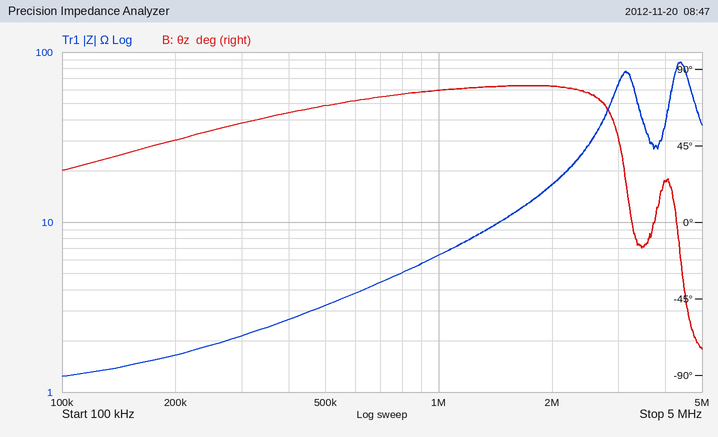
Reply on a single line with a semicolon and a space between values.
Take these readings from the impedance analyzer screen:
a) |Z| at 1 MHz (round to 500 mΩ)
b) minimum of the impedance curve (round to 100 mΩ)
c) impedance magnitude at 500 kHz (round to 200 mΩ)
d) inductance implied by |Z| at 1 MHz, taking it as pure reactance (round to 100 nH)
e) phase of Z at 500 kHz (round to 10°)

6.5 Ω; 1.2 Ω; 3.2 Ω; 1.0 µH; 70°
